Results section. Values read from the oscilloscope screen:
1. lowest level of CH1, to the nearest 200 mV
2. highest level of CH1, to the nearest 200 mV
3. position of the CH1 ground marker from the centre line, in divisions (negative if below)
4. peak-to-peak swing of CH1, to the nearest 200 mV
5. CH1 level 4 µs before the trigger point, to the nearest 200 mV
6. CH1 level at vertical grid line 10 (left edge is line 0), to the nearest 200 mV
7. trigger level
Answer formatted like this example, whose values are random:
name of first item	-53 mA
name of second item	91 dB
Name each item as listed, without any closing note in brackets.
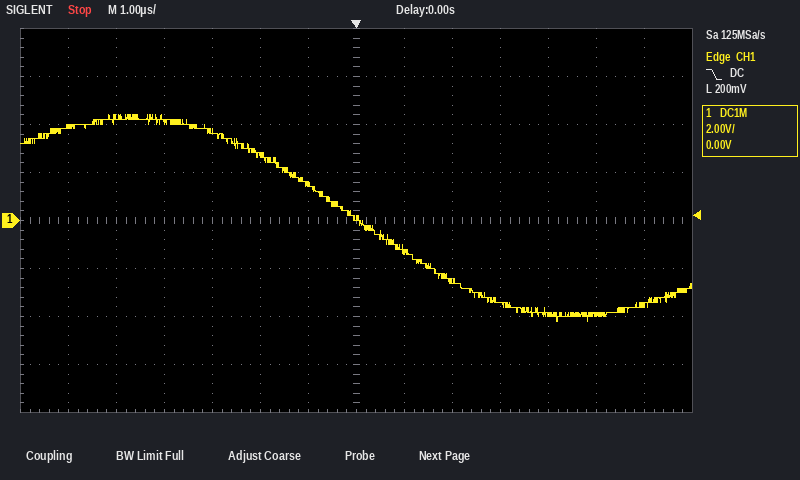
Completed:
lowest level of CH1, to the nearest 200 mV	-4.2 V
highest level of CH1, to the nearest 200 mV	4.4 V
position of the CH1 ground marker from the centre line, in divisions	0.0 div
peak-to-peak swing of CH1, to the nearest 200 mV	8.6 V
CH1 level 4 µs before the trigger point, to the nearest 200 mV	4.2 V
CH1 level at vertical grid line 10 (left edge is line 0), to the nearest 200 mV	-3.4 V
trigger level	200 mV
